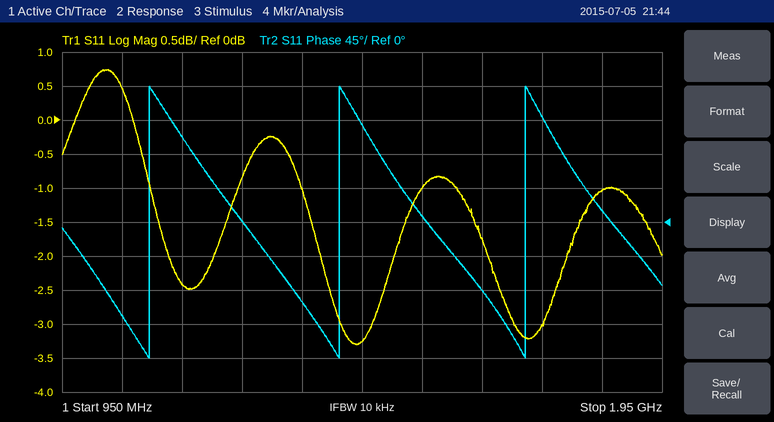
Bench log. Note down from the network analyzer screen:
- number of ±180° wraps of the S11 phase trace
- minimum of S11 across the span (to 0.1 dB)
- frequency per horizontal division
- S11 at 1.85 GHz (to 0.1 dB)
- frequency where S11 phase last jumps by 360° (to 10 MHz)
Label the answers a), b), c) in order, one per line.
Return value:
a) 3
b) -3.3 dB
c) 100 MHz
d) -1.0 dB
e) 1.72 GHz
